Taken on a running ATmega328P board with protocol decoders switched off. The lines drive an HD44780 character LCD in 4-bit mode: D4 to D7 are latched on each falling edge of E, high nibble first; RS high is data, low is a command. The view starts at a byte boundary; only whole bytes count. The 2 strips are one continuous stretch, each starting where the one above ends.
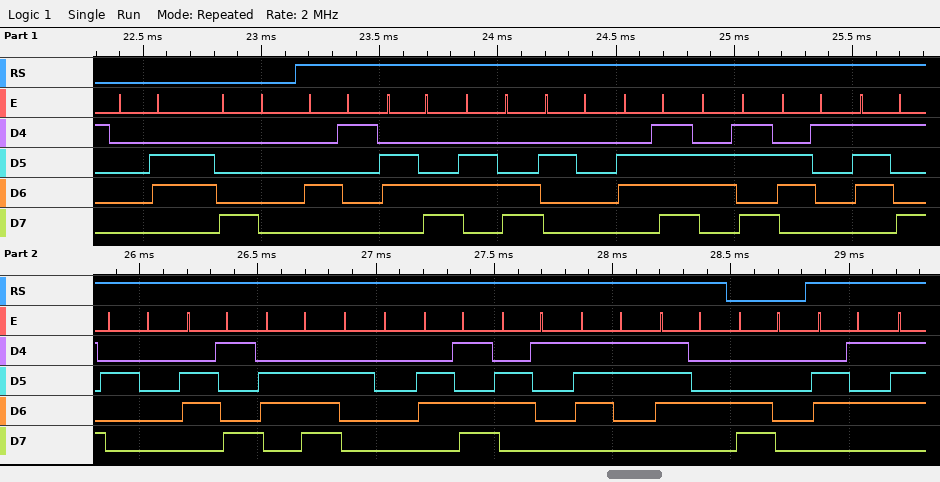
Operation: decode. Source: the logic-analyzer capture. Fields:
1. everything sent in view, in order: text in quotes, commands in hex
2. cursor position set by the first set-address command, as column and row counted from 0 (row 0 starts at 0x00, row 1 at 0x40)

0x06 0x80 "All okay in mast" 0xC0 "e"
column 0, row 0
